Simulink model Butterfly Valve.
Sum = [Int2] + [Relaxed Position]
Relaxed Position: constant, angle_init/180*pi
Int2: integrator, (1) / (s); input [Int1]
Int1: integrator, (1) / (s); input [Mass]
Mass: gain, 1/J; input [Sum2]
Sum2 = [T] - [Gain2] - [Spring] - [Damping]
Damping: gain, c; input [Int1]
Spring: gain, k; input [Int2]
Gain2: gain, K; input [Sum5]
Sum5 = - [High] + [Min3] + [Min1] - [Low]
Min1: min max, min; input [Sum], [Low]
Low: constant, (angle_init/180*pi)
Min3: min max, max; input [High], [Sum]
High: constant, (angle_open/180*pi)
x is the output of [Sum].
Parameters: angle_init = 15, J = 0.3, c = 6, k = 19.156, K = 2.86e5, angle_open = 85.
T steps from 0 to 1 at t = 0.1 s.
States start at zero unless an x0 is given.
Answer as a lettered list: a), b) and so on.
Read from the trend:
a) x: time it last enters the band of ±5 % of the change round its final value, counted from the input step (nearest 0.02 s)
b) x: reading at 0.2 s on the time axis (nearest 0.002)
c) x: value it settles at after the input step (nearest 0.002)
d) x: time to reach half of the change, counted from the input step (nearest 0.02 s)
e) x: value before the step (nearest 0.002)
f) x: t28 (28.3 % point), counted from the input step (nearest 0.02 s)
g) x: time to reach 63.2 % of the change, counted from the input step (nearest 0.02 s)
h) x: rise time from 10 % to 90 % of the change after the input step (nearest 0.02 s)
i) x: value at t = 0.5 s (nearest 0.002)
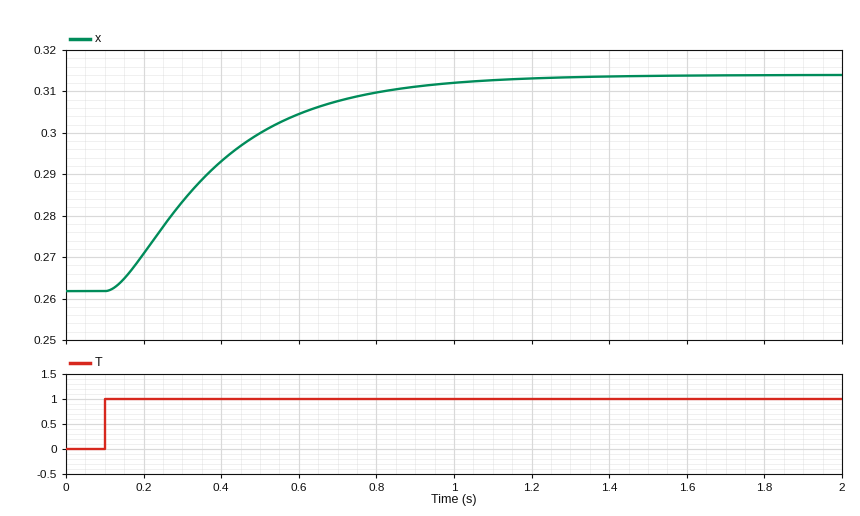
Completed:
a) 0.82 s
b) 0.270
c) 0.314
d) 0.24 s
e) 0.262
f) 0.14 s
g) 0.32 s
h) 0.58 s
i) 0.300
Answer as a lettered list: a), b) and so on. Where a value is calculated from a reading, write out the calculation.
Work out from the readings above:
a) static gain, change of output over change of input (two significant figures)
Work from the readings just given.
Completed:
a) (0.314 - 0.262) / (1 - 0) = 0.052
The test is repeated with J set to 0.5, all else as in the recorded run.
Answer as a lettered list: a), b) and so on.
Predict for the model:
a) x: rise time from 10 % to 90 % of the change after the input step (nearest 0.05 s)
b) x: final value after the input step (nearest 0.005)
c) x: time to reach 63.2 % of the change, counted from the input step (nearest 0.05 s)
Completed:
a) 0.50 s
b) 0.315
c) 0.35 s
